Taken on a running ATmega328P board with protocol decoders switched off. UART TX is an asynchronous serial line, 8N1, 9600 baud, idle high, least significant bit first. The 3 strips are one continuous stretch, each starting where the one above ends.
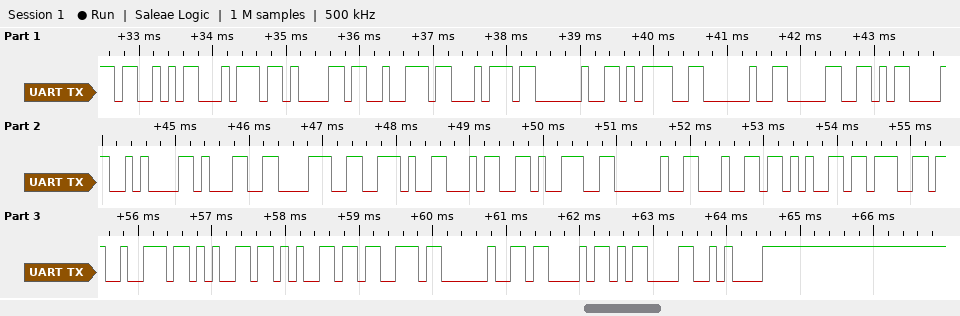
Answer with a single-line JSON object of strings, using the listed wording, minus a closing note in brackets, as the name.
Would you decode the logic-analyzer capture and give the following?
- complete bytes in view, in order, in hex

{"complete bytes in view, in order, in hex": "0x53 0x74 0x61 0x72 0x74 0x20 0x3D 0x20 0x30 0x0D 0x0A 0x31 0x38 0x2E 0x34 0x39 0x20 0x64 0x65 0x67 0x72 0x65 0x65 0x73 0x20 0x43 0x0D 0x0A"}
